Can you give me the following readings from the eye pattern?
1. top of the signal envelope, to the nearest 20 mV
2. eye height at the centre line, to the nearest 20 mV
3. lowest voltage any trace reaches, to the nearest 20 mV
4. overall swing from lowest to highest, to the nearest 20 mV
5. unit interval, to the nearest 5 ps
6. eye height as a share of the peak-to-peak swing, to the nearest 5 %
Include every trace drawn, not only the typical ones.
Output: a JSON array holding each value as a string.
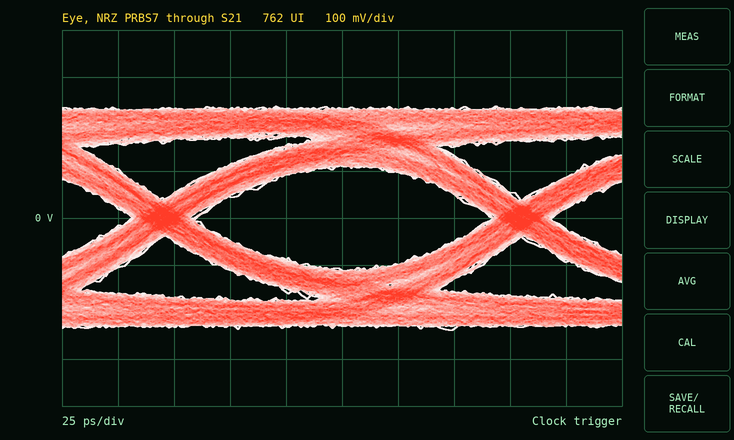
["240 mV", "220 mV", "-240 mV", "480 mV", "160 ps", "45 %"]
